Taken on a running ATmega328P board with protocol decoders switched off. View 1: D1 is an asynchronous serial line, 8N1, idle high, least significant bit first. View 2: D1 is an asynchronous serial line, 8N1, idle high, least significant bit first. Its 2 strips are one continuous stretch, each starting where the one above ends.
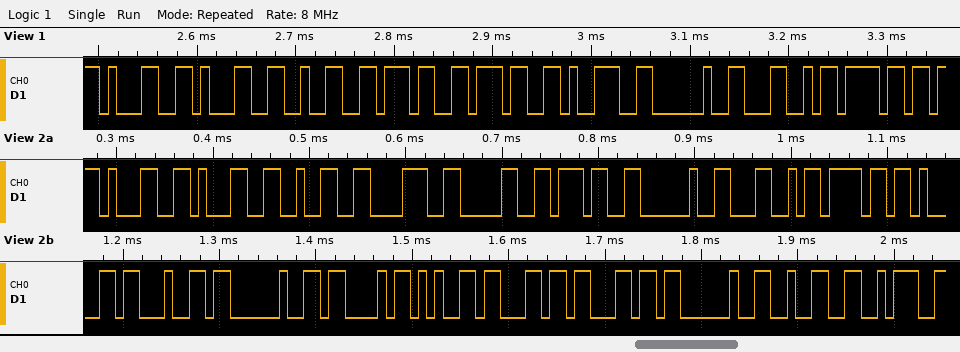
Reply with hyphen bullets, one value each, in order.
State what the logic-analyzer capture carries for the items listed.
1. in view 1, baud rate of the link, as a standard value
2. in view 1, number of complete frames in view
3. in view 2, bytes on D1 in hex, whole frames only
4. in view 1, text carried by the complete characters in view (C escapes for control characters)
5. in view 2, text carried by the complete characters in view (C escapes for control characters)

- 115200 baud
- 9
- 0x31 0x31 0x32 0x38 0x30 0x37 0x20 0x4C 0x6F 0x61 0x64 0x20 0x43 0x65 0x6C 0x6C 0x20 0x32 0x3A
- "112779 Lo"
- "112807 Load Cell 2:"
